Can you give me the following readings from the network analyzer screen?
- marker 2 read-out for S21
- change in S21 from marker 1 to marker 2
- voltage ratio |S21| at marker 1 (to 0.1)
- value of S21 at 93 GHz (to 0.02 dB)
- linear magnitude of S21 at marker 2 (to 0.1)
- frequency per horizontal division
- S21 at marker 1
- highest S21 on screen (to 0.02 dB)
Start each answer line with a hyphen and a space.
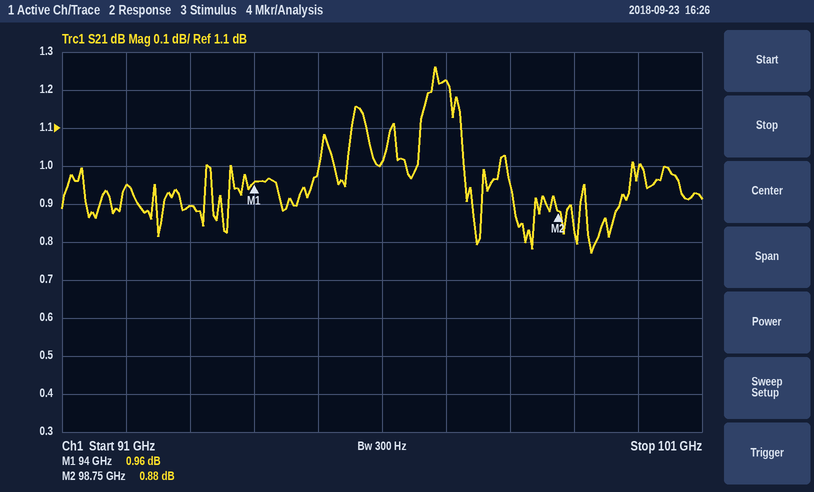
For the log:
- 0.88 dB
- -0.08 dB
- 1.1
- 0.90 dB
- 1.1
- 1 GHz
- 0.96 dB
- 1.26 dB
